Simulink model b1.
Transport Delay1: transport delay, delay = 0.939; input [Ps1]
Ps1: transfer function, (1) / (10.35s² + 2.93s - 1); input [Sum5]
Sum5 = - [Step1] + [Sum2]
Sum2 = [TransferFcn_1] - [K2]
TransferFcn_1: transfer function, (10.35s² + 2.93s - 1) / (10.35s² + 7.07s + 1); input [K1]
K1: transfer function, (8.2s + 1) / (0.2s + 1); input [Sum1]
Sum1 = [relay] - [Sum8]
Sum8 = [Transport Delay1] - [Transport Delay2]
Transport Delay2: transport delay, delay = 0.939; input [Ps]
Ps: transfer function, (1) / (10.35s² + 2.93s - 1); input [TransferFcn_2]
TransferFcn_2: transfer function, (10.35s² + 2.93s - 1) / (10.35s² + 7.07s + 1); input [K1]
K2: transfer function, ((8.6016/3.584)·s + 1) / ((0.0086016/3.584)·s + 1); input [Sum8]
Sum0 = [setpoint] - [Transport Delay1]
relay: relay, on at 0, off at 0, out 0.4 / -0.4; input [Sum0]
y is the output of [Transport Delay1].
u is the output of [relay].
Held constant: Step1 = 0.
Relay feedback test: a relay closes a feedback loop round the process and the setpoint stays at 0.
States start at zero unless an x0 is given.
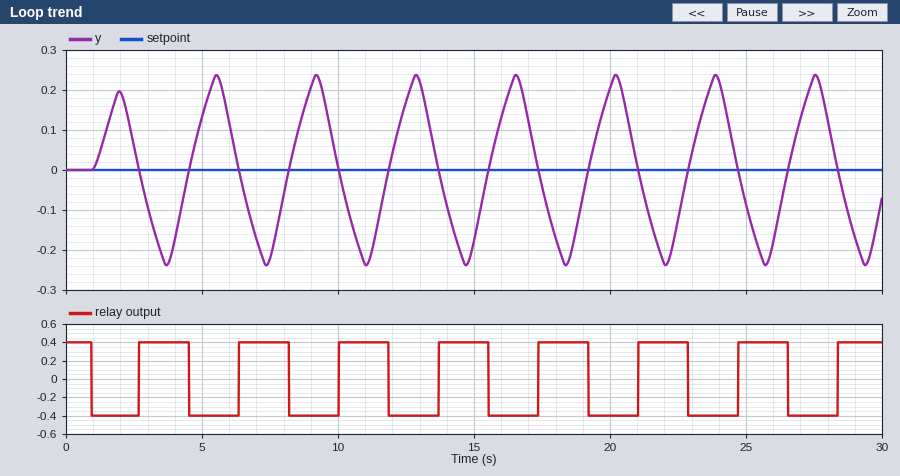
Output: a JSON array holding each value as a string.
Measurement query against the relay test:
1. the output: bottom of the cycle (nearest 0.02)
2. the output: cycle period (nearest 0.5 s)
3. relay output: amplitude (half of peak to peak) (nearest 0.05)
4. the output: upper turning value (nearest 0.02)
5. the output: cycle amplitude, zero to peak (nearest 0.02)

["-0.24", "3.5 s", "0.40", "0.24", "0.24"]
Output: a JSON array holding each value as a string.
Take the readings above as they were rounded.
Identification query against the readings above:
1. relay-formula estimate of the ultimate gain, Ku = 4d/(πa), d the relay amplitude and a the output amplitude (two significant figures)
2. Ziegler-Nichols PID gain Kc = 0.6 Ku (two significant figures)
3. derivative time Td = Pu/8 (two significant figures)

["2.1", "1.3", "0.44 s"]
